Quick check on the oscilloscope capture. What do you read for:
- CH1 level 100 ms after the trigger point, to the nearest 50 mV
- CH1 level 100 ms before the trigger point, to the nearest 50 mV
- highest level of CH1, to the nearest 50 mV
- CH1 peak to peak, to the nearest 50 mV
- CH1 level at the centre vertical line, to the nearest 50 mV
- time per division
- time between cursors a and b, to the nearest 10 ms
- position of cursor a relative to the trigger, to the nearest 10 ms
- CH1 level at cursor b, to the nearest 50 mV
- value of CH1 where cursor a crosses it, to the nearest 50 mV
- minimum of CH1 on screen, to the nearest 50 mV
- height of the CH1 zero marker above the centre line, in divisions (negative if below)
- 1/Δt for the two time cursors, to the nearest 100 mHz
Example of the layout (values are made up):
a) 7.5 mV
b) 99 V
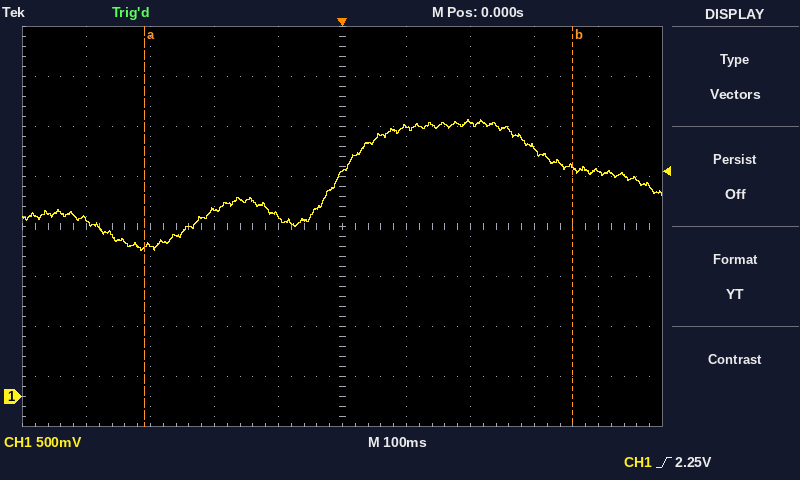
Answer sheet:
a) 2.70 V
b) 1.80 V
c) 2.75 V
d) 1.30 V
e) 2.25 V
f) 100 ms
g) 670 ms
h) -310 ms
i) 2.30 V
j) 1.50 V
k) 1.45 V
l) -3.4 div
m) 1.5 Hz
